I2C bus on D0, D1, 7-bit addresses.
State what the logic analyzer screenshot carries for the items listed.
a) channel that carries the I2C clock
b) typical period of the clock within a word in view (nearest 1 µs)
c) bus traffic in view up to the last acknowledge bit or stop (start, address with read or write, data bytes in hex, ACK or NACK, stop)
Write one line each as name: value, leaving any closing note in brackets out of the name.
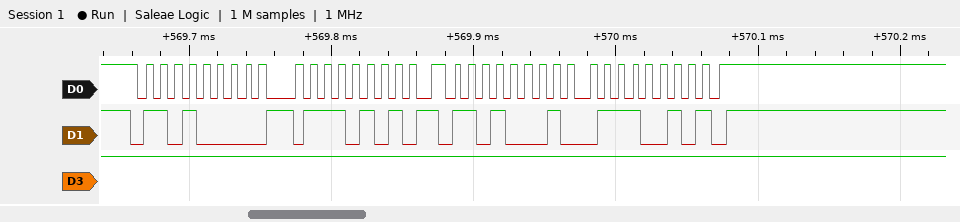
channel that carries the I2C clock: D0
typical period of the clock within a word in view: 10 µs
bus traffic in view up to the last acknowledge bit or stop: start, address 68 write ACK, 75 ACK, repeated start, address 68 read ACK, 72 NACK, stop
